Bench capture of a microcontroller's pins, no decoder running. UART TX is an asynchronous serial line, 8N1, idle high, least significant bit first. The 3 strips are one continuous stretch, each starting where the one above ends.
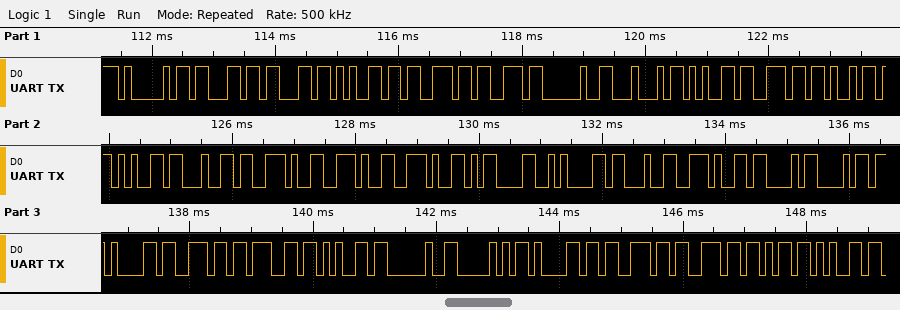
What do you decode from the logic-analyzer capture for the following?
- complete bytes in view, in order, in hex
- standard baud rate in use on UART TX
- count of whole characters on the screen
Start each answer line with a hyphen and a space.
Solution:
- 41 63 63 65 73 73 20 44 65 6E 69 65 64 2E 2E 2E 0D 0A 23 2E 43 68 61 6E 67 65 20 50 61 73 73 6B 65
- 9600 baud
- 33
